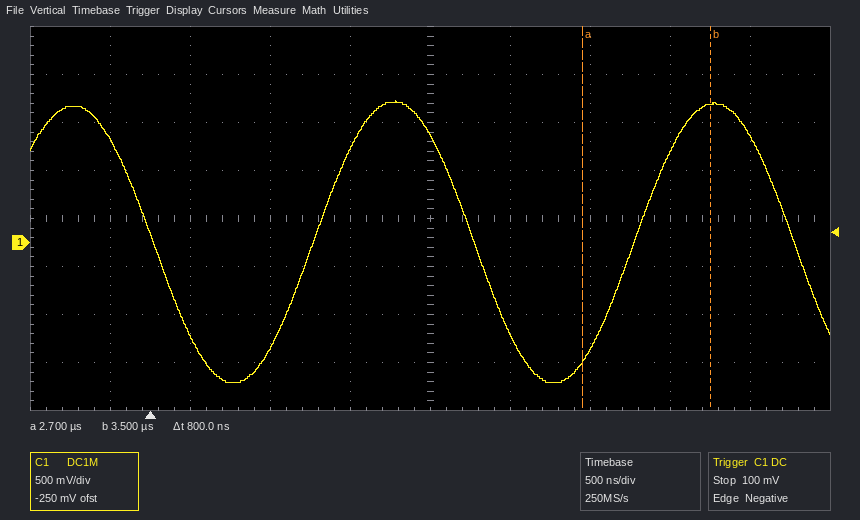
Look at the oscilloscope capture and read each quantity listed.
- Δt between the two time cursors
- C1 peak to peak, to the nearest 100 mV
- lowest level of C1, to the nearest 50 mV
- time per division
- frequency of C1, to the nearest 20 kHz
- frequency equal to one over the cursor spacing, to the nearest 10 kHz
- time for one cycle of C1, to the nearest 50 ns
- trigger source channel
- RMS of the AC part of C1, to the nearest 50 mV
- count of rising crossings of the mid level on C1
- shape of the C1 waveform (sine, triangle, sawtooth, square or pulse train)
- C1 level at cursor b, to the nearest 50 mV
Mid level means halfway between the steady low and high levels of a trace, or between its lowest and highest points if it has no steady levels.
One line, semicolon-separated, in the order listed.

800 ns; 2.90 V; -1.45 V; 500 ns; 500 kHz; 1.25 MHz; 2.00 µs; C1; 1.05 V; 2; sine; 1.45 V
